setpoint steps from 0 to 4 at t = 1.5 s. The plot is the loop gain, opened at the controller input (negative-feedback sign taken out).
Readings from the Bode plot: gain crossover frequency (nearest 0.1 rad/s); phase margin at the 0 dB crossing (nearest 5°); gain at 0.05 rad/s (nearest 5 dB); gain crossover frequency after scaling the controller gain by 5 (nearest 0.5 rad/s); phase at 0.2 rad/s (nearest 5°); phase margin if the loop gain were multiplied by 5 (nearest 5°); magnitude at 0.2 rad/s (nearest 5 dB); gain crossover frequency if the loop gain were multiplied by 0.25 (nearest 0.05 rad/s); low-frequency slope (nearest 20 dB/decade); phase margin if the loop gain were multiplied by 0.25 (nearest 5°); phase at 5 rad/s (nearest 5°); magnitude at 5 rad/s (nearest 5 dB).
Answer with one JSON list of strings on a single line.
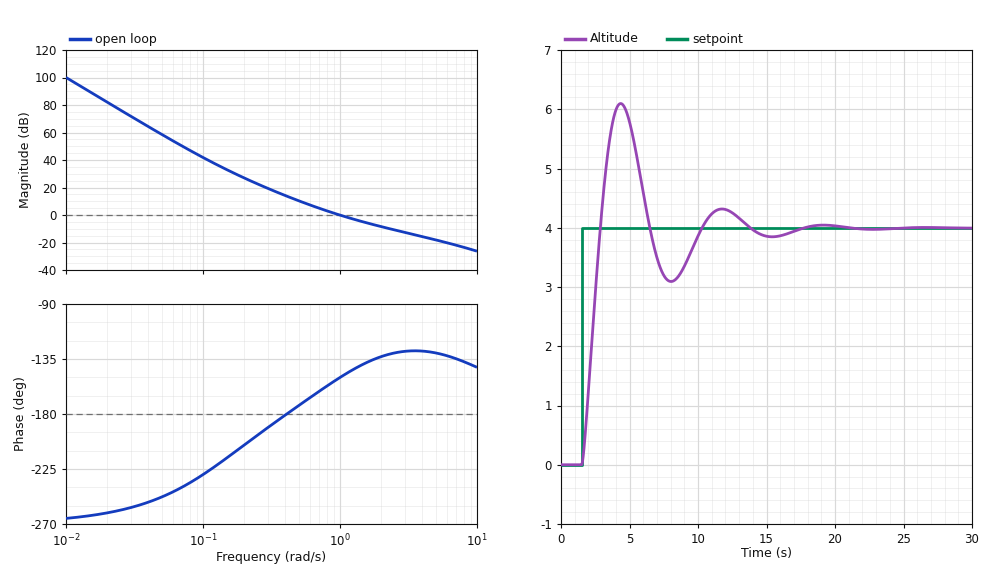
["1.0 rad/s", "30°", "60 dB", "3.5 rad/s", "-205°", "50°", "25 dB", "0.45 rad/s", "-60 dB/decade", "5°", "-130°", "-20 dB"]
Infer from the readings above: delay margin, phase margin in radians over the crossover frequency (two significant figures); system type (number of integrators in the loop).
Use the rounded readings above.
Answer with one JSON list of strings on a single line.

["0.52 s", "3"]
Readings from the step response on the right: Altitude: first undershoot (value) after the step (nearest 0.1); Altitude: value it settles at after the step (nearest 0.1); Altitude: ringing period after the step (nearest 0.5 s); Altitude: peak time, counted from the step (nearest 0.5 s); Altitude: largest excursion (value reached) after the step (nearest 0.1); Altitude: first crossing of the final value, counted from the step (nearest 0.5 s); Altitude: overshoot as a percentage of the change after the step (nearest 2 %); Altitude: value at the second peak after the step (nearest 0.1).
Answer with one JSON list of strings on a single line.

["3.1", "4.0", "7.5 s", "3.0 s", "6.1", "1.5 s", "52 %", "4.3"]
